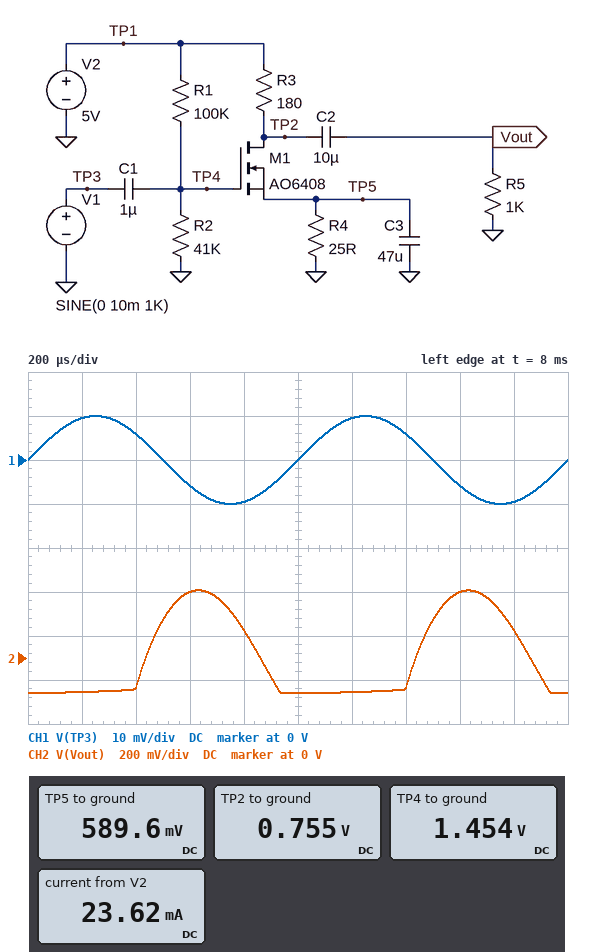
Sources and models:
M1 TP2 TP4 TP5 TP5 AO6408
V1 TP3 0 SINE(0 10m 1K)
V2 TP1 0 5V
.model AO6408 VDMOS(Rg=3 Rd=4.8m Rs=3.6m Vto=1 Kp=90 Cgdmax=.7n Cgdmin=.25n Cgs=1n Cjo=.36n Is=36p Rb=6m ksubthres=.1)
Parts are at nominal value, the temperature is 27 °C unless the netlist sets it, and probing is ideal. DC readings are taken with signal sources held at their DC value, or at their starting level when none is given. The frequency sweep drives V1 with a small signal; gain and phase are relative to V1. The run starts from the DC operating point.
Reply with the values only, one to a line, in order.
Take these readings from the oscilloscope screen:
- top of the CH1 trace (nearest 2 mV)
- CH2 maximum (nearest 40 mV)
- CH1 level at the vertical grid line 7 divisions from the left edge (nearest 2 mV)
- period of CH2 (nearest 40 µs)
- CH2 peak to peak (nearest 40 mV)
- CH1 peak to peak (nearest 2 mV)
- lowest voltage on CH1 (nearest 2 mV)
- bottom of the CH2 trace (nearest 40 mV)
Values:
10 mV
320 mV
6 mV
1.00 ms
480 mV
20 mV
-10 mV
-160 mV
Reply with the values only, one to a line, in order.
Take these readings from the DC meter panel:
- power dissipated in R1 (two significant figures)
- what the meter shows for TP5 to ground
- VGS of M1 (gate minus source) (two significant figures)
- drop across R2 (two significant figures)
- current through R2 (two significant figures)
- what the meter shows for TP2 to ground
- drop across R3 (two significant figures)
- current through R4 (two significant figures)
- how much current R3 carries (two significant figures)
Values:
130 µW
589.6 mV
860 mV
1.5 V
35 µA
0.755 V
4.2 V
24 mA
24 mA
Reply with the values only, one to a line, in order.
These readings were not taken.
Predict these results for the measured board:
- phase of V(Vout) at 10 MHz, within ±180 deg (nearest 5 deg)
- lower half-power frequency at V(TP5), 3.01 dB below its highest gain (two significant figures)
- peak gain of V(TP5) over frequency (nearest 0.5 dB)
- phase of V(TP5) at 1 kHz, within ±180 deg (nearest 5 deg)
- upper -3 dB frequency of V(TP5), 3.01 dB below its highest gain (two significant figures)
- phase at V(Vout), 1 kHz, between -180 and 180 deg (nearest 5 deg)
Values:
80 deg
5.4 Hz
-1.0 dB
-35 deg
1.5 kHz
-130 deg
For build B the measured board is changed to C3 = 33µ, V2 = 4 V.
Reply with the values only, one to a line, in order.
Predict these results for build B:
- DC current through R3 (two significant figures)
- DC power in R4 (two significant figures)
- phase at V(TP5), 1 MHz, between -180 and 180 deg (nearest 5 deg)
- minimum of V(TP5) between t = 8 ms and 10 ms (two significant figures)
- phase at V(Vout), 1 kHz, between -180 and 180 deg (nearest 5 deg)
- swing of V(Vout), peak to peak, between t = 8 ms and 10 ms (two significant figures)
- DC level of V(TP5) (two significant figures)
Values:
13 mA
4.4 mW
-110 deg
320 mV
-135 deg
440 mV
330 mV
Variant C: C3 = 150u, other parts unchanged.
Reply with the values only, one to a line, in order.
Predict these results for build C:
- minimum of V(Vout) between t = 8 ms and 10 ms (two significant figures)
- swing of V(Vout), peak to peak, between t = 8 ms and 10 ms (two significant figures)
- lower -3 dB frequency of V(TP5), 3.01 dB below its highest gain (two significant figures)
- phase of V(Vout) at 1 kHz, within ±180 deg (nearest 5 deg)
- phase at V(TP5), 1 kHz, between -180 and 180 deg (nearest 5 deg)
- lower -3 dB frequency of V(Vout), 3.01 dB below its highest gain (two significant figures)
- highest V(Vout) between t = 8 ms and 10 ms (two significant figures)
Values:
-170 mV
550 mV
5.3 Hz
-155 deg
-65 deg
470 Hz
380 mV
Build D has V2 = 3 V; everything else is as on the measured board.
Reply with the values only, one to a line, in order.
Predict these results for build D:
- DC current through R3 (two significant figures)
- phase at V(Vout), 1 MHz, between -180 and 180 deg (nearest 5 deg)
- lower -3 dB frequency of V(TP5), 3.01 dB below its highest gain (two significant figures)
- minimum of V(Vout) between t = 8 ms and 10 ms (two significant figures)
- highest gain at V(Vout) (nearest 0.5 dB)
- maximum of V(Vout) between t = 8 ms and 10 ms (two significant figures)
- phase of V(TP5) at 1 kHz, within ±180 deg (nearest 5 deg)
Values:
4.1 mA
145 deg
5.3 Hz
-120 mV
21.5 dB
110 mV
-70 deg
